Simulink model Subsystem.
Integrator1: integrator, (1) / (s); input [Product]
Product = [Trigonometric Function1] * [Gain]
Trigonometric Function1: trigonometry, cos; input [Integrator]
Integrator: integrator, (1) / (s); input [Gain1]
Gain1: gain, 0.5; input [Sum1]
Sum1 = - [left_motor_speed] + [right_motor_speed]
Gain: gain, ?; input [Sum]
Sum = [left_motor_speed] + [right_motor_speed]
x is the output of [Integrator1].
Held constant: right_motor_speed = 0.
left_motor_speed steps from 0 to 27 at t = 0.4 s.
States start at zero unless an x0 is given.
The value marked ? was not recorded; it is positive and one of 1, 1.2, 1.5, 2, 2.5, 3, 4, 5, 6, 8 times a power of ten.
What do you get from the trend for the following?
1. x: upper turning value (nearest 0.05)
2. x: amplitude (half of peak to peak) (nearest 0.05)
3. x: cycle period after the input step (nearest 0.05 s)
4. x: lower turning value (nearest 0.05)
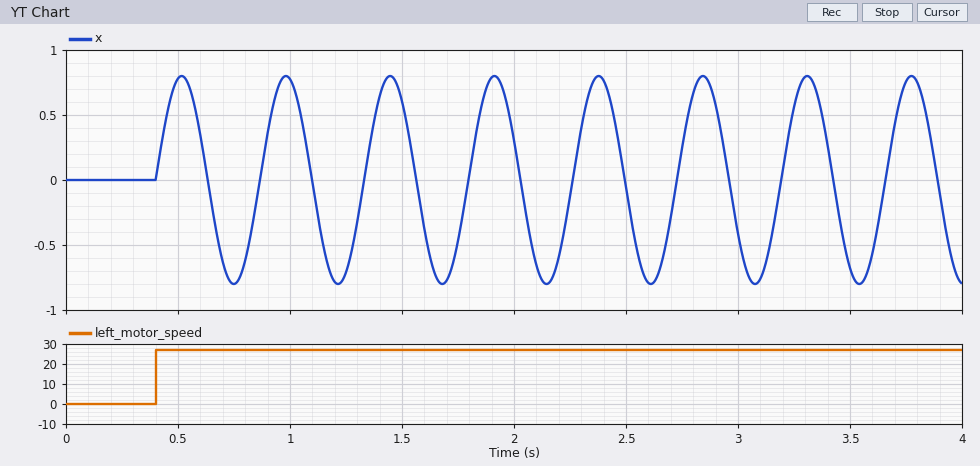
0.80
0.80
0.45 s
-0.80
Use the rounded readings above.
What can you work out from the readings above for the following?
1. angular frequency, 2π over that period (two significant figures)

14 rad/s
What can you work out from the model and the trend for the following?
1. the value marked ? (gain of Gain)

0.4
